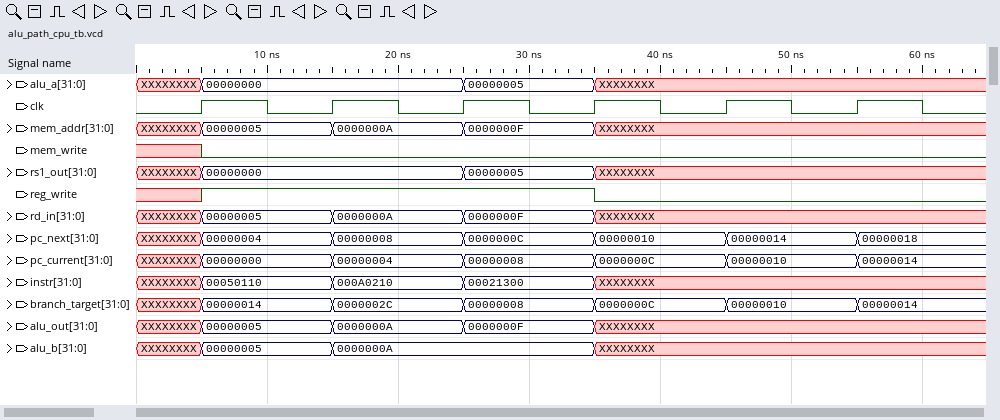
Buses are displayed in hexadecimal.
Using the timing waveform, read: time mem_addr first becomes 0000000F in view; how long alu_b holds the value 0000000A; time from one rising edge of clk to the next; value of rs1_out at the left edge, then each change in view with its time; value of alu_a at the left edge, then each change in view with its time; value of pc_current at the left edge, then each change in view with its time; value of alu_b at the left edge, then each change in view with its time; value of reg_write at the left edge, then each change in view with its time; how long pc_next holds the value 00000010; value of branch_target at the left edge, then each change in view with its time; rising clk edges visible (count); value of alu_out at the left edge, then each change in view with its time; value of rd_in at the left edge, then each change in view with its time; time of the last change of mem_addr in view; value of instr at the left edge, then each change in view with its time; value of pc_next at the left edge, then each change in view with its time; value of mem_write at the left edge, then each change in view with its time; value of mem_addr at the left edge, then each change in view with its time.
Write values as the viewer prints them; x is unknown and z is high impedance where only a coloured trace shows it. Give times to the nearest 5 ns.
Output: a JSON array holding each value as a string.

["25 ns", "20 ns", "10 ns", "XXXXXXXX, 00000000 at 5 ns, 00000005 at 25 ns, XXXXXXXX at 35 ns", "XXXXXXXX, 00000000 at 5 ns, 00000005 at 25 ns, XXXXXXXX at 35 ns", "XXXXXXXX, 00000000 at 5 ns, 00000004 at 15 ns, 00000008 at 25 ns, 0000000C at 35 ns, 00000010 at 45 ns, 00000014 at 55 ns", "XXXXXXXX, 00000005 at 5 ns, 0000000A at 15 ns, XXXXXXXX at 35 ns", "x, 1 at 5 ns, 0 at 35 ns", "10 ns", "XXXXXXXX, 00000014 at 5 ns, 0000002C at 15 ns, 00000008 at 25 ns, 0000000C at 35 ns, 00000010 at 45 ns, 00000014 at 55 ns", "6", "XXXXXXXX, 00000005 at 5 ns, 0000000A at 15 ns, 0000000F at 25 ns, XXXXXXXX at 35 ns", "XXXXXXXX, 00000005 at 5 ns, 0000000A at 15 ns, 0000000F at 25 ns, XXXXXXXX at 35 ns", "35 ns", "XXXXXXXX, 00050110 at 5 ns, 000A0210 at 15 ns, 00021300 at 25 ns, XXXXXXXX at 35 ns", "XXXXXXXX, 00000004 at 5 ns, 00000008 at 15 ns, 0000000C at 25 ns, 00000010 at 35 ns, 00000014 at 45 ns, 00000018 at 55 ns", "x, 0 at 5 ns", "XXXXXXXX, 00000005 at 5 ns, 0000000A at 15 ns, 0000000F at 25 ns, XXXXXXXX at 35 ns"]
